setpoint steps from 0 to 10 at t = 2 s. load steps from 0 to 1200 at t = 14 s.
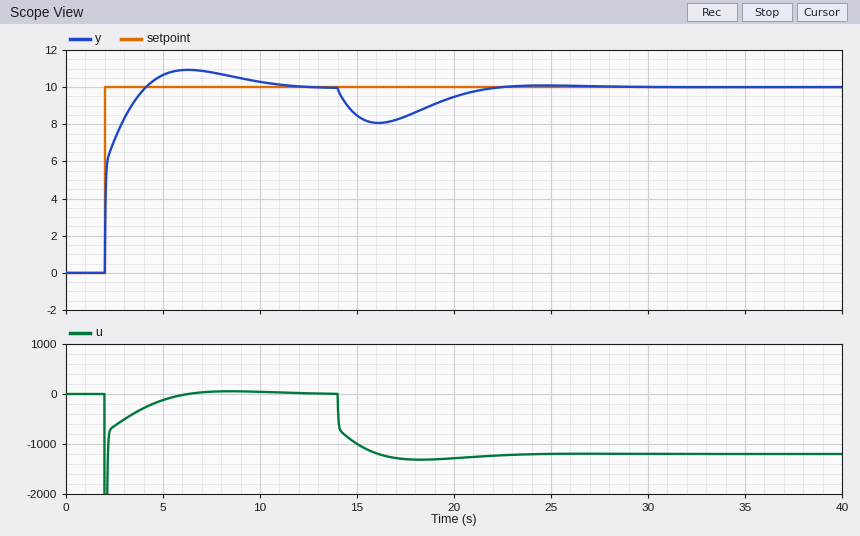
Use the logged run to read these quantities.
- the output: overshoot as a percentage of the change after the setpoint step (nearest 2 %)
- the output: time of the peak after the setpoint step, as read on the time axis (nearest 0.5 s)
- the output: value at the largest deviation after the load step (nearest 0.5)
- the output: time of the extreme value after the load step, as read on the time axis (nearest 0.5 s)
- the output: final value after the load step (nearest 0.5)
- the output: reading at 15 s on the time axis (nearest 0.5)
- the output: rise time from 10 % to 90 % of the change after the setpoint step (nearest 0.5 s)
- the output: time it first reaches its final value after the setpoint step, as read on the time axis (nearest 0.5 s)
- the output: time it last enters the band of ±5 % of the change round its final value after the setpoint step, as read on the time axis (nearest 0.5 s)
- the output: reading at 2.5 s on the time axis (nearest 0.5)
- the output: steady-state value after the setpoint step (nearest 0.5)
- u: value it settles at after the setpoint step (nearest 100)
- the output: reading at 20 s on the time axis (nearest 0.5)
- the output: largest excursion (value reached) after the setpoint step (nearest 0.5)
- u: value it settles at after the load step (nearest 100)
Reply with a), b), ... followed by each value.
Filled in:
a) 10 %
b) 6.5 s
c) 8.0
d) 16.0 s
e) 10.0
f) 8.5
g) 1.5 s
h) 4.0 s
i) 9.0 s
j) 7.0
k) 10.0
l) 0
m) 9.5
n) 11.0
o) -1200
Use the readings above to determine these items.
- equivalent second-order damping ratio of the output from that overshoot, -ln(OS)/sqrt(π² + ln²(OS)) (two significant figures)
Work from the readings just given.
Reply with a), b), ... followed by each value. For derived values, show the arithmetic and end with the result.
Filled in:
a) ln(0.1) = -2.303; 2.303 / sqrt(9.870 + 5.302) = 0.59
